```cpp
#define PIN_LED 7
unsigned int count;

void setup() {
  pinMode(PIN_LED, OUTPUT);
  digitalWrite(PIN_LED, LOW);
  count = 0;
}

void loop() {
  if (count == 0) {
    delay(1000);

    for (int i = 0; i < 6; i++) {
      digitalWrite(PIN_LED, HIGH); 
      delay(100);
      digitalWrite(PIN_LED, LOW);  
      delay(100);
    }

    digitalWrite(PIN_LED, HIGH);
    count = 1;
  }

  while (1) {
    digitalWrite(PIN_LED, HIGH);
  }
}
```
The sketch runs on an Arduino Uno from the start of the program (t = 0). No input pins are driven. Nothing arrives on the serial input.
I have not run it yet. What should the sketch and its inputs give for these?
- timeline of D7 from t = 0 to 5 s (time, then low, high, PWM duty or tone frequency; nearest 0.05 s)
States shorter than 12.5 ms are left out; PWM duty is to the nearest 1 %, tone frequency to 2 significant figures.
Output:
0 s low; 1 s high; 1.1 s low; 1.2 s high; 1.3 s low; 1.4 s high; 1.5 s low; 1.6 s high; 1.7 s low; 1.8 s high; 1.9 s low; 2 s high; 2.1 s low; 2.2 s high
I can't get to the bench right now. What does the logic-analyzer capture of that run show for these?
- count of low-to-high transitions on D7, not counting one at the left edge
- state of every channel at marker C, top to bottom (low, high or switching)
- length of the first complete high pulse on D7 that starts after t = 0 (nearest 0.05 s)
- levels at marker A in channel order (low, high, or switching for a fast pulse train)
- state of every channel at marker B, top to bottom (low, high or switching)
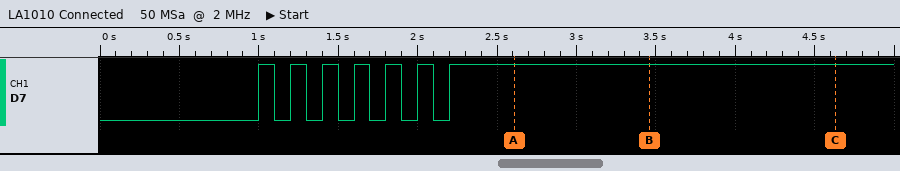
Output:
7
D7 high
0.10 s
D7 high
D7 high
